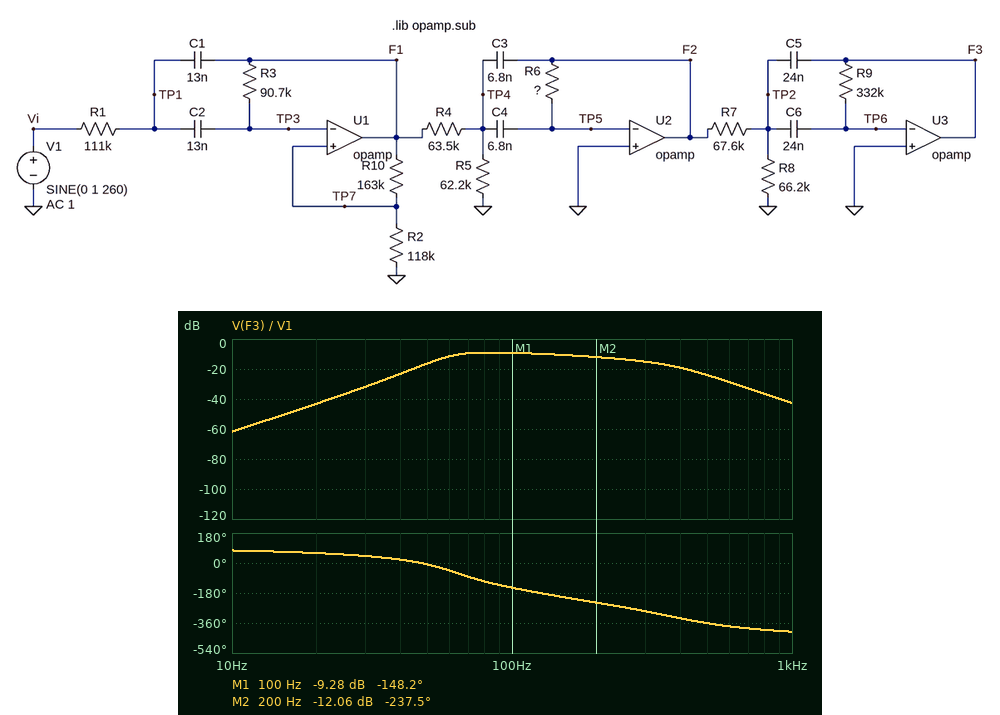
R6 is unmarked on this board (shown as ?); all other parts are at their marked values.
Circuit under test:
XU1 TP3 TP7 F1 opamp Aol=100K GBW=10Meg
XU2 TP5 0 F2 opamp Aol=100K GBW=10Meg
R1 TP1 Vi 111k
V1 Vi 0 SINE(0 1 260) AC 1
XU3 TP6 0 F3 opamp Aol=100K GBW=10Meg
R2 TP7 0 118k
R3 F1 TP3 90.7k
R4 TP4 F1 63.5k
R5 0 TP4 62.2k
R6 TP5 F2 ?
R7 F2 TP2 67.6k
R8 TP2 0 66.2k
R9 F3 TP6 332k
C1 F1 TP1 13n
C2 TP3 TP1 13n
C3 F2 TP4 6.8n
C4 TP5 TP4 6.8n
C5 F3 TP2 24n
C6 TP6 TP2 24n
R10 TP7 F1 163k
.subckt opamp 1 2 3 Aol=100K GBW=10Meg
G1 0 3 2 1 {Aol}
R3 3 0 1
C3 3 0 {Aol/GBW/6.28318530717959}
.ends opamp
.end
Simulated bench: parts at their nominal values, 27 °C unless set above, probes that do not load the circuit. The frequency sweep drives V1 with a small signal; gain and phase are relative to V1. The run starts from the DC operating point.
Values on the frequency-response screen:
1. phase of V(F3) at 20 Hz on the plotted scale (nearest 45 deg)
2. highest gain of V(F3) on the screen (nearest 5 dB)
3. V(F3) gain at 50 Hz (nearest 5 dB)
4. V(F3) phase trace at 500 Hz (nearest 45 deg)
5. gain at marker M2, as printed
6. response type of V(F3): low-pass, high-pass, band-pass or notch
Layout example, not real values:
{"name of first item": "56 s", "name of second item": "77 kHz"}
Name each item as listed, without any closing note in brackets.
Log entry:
{"phase of V(F3) at 20 Hz on the plotted scale": "45 deg", "highest gain of V(F3) on the screen": "-10 dB", "V(F3) gain at 50 Hz": "-15 dB", "V(F3) phase trace at 500 Hz": "-360 deg", "gain at marker M2, as printed": "-12.06 dB", "response type of V(F3): low-pass, high-pass, band-pass or notch": "band-pass"}
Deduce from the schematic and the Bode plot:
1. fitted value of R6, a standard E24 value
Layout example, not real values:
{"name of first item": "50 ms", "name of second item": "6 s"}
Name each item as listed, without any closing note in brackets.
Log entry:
{"fitted value of R6, a standard E24 value": "120 kΩ"}
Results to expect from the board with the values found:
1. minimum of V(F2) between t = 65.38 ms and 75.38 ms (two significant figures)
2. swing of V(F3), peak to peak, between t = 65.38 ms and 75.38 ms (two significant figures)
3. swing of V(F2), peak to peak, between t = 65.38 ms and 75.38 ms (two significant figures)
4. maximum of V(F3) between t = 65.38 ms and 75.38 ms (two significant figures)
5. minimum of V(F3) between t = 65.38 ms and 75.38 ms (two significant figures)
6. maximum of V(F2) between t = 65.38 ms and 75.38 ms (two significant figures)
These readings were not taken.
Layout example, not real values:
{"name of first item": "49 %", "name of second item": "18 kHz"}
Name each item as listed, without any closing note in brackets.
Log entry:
{"minimum of V(F2) between t = 65.38 ms and 75.38 ms": "-510 mV", "swing of V(F3), peak to peak, between t = 65.38 ms and 75.38 ms": "410 mV", "swing of V(F2), peak to peak, between t = 65.38 ms and 75.38 ms": "1.0 V", "maximum of V(F3) between t = 65.38 ms and 75.38 ms": "200 mV", "minimum of V(F3) between t = 65.38 ms and 75.38 ms": "-200 mV", "maximum of V(F2) between t = 65.38 ms and 75.38 ms": "510 mV"}
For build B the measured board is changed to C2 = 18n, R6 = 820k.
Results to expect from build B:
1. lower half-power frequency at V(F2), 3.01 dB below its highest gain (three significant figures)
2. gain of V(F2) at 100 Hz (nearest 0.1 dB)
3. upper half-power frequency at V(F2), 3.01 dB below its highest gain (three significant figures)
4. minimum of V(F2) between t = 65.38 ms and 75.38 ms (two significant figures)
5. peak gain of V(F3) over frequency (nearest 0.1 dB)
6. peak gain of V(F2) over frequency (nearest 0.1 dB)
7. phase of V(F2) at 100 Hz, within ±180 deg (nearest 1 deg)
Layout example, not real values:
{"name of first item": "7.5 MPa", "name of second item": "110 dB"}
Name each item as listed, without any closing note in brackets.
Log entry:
{"lower half-power frequency at V(F2), 3.01 dB below its highest gain": "116 Hz", "gain of V(F2) at 100 Hz": "11.2 dB", "upper half-power frequency at V(F2), 3.01 dB below its highest gain": "170 Hz", "minimum of V(F2) between t = 65.38 ms and 75.38 ms": "-1.4 V", "peak gain of V(F3) over frequency": "15.7 dB", "peak gain of V(F2) over frequency": "17.3 dB", "phase of V(F2) at 100 Hz, within ±180 deg": "66 deg"}
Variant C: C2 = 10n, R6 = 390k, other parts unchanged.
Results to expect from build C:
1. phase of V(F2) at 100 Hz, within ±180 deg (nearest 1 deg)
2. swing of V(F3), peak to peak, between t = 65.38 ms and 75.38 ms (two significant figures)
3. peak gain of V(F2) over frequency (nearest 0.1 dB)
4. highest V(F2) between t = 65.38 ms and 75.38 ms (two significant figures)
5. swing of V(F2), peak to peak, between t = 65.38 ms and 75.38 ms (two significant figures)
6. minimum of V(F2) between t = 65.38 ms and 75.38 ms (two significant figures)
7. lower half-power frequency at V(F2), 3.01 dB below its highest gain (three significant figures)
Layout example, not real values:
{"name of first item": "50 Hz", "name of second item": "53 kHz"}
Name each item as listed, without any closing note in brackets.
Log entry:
{"phase of V(F2) at 100 Hz, within ±180 deg": "93 deg", "swing of V(F3), peak to peak, between t = 65.38 ms and 75.38 ms": "1.3 V", "peak gain of V(F2) over frequency": "7.1 dB", "highest V(F2) between t = 65.38 ms and 75.38 ms": "1.6 V", "swing of V(F2), peak to peak, between t = 65.38 ms and 75.38 ms": "3.2 V", "minimum of V(F2) between t = 65.38 ms and 75.38 ms": "-1.6 V", "lower half-power frequency at V(F2), 3.01 dB below its highest gain": "151 Hz"}
